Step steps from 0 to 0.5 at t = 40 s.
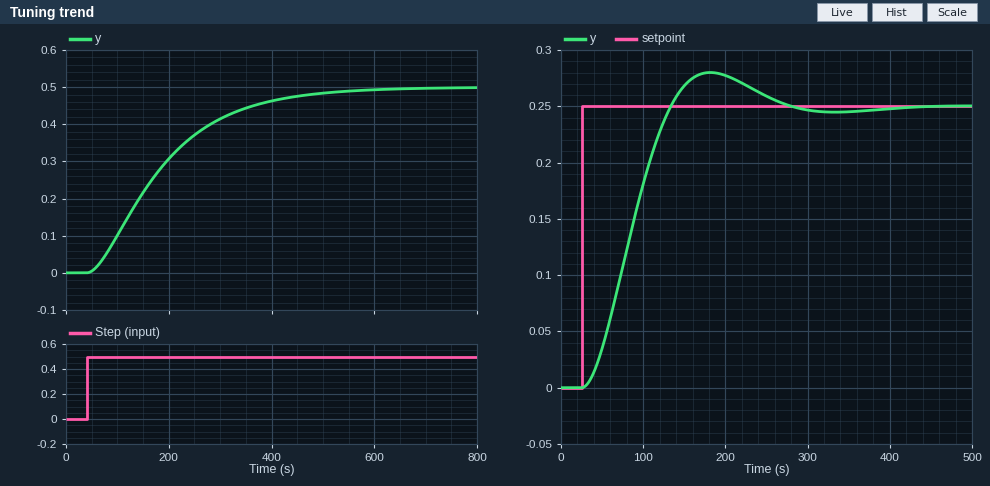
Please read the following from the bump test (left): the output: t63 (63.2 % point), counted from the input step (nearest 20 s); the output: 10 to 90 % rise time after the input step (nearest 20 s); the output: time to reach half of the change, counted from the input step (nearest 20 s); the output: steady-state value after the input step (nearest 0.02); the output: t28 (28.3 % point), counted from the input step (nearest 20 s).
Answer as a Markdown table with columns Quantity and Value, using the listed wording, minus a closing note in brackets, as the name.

| Quantity | Value |
|---|---|
| the output: t63 (63.2 % point), counted from the input step | 160 s |
| the output: 10 to 90 % rise time after the input step | 280 s |
| the output: time to reach half of the change, counted from the input step | 120 s |
| the output: steady-state value after the input step | 0.50 |
| the output: t28 (28.3 % point), counted from the input step | 80 s |
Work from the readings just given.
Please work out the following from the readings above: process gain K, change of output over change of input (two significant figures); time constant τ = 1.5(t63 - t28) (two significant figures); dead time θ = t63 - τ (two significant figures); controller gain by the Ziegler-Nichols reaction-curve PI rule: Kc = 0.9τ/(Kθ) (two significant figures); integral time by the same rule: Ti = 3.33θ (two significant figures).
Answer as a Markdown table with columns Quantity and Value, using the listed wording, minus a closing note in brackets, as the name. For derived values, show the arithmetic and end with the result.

| Quantity | Value |
|---|---|
| process gain K, change of output over change of input | (0.5 - 0) / 0.5 = 1.0 |
| time constant τ = 1.5(t63 - t28) | 1.5 × (160 - 80) = 120 s |
| dead time θ = t63 - τ | 160 - 120 = 40 s |
| controller gain by the Ziegler-Nichols reaction-curve PI rule: Kc = 0.9τ/(Kθ) | 0.9 × 120 / (1 × 40) = 2.7 |
| integral time by the same rule: Ti = 3.33θ | 3.33 × 40 = 130 s |
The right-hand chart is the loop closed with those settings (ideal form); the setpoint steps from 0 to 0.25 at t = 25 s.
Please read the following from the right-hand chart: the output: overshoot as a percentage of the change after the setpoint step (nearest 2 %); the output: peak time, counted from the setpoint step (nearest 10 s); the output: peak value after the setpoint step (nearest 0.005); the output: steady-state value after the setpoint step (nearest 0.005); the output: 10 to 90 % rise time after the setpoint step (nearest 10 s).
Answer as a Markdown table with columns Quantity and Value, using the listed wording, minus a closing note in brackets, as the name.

| Quantity | Value |
|---|---|
| the output: overshoot as a percentage of the change after the setpoint step | 12 % |
| the output: peak time, counted from the setpoint step | 160 s |
| the output: peak value after the setpoint step | 0.280 |
| the output: steady-state value after the setpoint step | 0.250 |
| the output: 10 to 90 % rise time after the setpoint step | 70 s |
